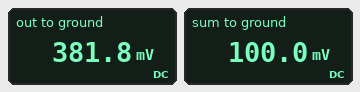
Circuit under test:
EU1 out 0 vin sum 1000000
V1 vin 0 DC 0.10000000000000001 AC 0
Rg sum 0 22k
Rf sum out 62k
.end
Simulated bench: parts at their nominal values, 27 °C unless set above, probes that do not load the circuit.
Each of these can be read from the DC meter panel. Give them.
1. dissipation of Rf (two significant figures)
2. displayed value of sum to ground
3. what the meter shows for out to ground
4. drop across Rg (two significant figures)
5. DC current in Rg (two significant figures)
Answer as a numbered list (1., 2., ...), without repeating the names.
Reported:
1. 1.3 µW
2. 100.0 mV
3. 381.8 mV
4. 100 mV
5. 4.5 µA
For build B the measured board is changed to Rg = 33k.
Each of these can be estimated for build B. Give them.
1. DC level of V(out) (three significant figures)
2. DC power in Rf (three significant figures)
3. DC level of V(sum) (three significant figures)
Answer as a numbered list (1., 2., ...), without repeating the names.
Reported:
1. 288 mV
2. 569 nW
3. 100 mV
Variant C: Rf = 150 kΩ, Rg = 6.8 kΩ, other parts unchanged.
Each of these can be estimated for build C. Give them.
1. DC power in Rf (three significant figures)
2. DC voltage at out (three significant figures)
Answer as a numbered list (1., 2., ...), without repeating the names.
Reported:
1. 32.4 µW
2. 2.31 V
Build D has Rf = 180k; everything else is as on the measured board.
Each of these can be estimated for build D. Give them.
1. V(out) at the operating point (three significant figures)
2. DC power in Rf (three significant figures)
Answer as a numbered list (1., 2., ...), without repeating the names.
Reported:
1. 918 mV
2. 3.72 µW
